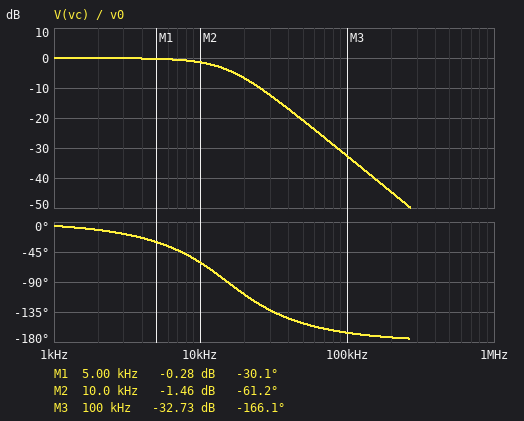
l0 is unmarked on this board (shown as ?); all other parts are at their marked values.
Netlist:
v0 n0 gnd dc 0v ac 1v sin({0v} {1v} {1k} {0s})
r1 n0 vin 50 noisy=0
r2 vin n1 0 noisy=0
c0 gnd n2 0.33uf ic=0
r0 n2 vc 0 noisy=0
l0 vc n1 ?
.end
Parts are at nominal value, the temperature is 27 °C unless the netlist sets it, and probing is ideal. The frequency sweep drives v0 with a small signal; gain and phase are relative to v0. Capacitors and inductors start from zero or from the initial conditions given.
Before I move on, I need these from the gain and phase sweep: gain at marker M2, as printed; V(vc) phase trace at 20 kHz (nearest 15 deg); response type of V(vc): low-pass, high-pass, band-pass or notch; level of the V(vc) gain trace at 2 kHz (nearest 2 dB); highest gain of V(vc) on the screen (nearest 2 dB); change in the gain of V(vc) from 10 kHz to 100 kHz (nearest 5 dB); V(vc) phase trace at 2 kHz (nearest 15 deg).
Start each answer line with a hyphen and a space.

- -1.46 dB
- -105 deg
- low-pass
- 0 dB
- 0 dB
- -30 dB
- -15 deg
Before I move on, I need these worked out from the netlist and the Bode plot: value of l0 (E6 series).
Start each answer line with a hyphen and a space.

- 330 µH
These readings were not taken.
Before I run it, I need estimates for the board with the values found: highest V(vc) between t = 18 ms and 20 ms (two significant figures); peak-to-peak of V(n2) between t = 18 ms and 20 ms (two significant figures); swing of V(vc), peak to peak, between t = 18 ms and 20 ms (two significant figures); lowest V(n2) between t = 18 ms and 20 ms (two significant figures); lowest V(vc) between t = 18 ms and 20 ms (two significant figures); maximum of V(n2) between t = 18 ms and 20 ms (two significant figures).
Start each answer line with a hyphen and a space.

- 1.0 V
- 2.0 V
- 2.0 V
- -1.0 V
- -1.0 V
- 1.0 V
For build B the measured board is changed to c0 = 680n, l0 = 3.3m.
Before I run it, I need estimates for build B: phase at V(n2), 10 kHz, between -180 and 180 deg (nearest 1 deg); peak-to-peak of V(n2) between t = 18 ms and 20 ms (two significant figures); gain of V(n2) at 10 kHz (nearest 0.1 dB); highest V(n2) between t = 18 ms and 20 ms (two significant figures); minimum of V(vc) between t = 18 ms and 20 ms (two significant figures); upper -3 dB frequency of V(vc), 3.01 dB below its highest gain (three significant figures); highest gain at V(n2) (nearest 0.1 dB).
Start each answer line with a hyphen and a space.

- -165 deg
- 2.1 V
- -18.2 dB
- 1.1 V
- -1.1 V
- 3.99 kHz
- 3.5 dB
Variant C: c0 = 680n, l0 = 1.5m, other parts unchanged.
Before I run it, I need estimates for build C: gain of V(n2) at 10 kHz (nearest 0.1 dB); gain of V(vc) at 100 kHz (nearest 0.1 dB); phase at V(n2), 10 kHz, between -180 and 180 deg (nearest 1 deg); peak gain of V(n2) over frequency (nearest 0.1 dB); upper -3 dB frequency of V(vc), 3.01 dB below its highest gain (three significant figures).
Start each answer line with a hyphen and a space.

- -11.4 dB
- -52.1 dB
- -145 deg
- 0.9 dB
- 5.76 kHz
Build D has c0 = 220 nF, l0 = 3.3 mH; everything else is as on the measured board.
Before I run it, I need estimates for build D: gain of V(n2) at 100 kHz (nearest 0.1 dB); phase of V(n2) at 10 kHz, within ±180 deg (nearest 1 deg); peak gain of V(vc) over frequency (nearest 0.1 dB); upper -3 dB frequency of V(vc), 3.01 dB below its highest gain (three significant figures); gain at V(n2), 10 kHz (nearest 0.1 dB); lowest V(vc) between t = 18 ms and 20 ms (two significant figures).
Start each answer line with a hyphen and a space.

- -49.1 dB
- -160 deg
- 8.0 dB
- 6.78 kHz
- -6.0 dB
- -1.0 V
